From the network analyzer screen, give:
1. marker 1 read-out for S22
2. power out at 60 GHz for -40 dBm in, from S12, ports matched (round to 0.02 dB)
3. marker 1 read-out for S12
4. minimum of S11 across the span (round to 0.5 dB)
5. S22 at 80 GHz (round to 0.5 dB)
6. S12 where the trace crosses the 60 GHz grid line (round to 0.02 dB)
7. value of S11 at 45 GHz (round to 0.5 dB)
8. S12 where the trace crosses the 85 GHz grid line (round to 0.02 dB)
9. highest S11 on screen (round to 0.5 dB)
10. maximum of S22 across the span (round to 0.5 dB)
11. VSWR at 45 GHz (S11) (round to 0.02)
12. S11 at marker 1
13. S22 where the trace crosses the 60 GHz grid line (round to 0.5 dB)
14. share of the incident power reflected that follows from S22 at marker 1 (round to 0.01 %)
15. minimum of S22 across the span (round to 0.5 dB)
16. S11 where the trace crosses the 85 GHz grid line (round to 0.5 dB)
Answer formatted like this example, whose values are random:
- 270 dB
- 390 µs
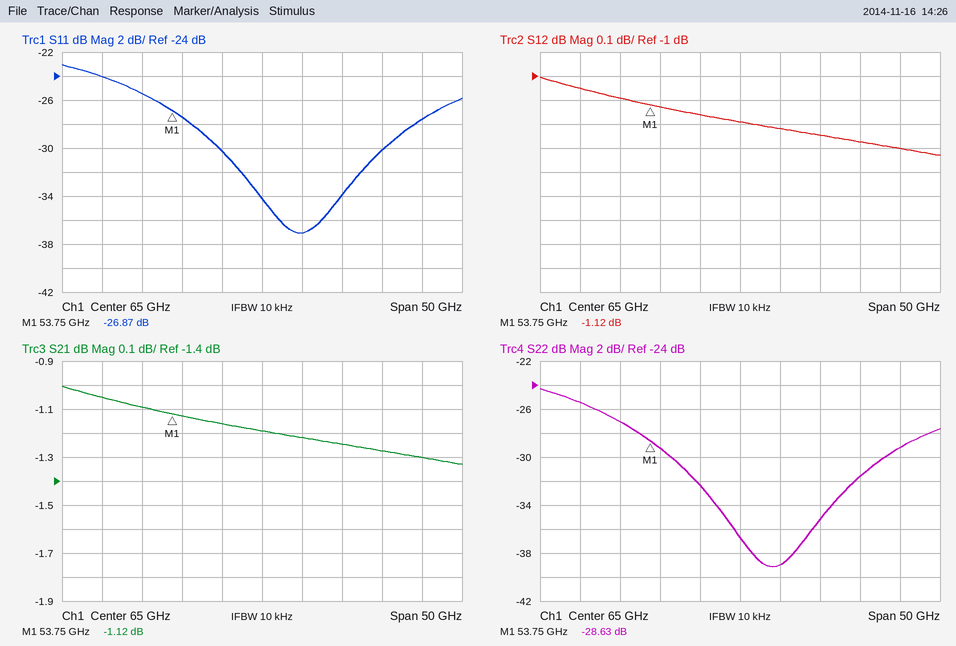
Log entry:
- -28.63 dB
- -41.16 dBm
- -1.12 dB
- -37.0 dB
- -31.5 dB
- -1.16 dB
- -24.0 dB
- -1.30 dB
- -23.0 dB
- -24.5 dB
- 1.14
- -26.87 dB
- -32.5 dB
- 0.14 %
- -39.0 dB
- -27.5 dB
